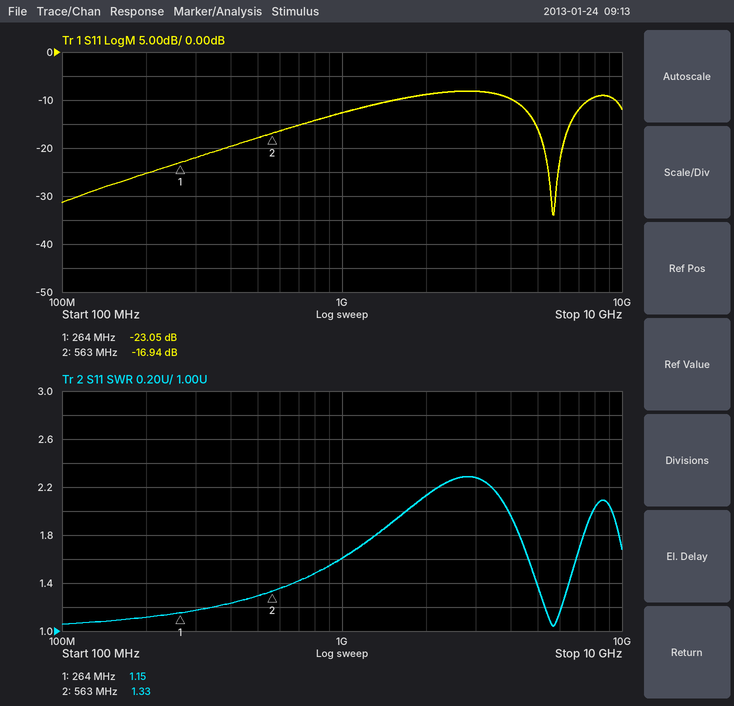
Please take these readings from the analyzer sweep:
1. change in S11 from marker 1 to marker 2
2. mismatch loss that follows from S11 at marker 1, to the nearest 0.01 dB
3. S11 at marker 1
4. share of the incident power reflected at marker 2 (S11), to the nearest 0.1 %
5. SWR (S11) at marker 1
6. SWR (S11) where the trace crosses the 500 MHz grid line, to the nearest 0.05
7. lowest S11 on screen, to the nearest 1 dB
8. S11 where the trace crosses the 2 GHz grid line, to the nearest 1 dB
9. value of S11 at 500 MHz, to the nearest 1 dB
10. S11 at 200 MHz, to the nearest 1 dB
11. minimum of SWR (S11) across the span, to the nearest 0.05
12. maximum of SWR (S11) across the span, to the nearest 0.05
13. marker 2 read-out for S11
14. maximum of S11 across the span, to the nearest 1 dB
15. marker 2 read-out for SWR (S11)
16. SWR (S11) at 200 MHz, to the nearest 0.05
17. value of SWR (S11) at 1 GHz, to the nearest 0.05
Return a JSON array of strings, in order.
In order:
["6.11 dB", "0.02 dB", "-23.05 dB", "2.0 %", "1.15", "1.30", "-34 dB", "-9 dB", "-18 dB", "-25 dB", "1.05", "2.30", "-16.94 dB", "-8 dB", "1.33", "1.10", "1.60"]
